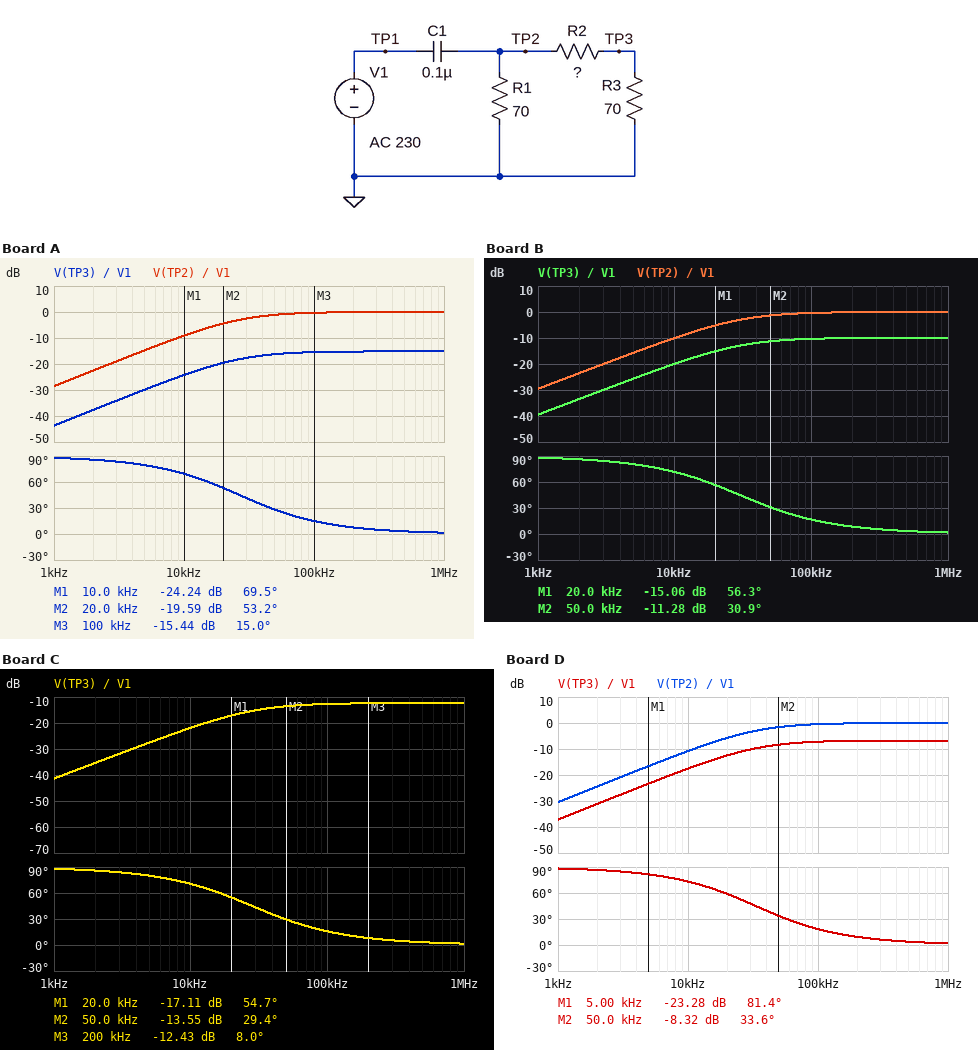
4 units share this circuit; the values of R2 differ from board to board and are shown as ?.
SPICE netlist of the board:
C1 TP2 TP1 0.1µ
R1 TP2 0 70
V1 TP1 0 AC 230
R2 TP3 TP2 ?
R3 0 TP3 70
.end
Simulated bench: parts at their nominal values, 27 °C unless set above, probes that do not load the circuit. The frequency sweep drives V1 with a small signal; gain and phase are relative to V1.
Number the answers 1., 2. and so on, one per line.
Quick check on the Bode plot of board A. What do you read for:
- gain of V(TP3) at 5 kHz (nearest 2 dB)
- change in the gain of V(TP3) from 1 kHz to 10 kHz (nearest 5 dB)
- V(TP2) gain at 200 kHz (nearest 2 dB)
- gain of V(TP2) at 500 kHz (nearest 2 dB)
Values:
1. -30 dB
2. 20 dB
3. 0 dB
4. 0 dB
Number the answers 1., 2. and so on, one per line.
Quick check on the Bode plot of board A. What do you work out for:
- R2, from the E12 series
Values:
1. 330 Ω
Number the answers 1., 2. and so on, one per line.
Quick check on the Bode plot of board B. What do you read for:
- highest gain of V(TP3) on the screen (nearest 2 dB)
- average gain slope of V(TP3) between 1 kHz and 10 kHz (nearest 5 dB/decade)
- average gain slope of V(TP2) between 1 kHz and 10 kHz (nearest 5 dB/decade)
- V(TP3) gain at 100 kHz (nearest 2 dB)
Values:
1. -10 dB
2. 20 dB/decade
3. 20 dB/decade
4. -10 dB
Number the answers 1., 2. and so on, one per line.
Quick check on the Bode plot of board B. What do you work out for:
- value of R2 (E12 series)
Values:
1. 150 Ω
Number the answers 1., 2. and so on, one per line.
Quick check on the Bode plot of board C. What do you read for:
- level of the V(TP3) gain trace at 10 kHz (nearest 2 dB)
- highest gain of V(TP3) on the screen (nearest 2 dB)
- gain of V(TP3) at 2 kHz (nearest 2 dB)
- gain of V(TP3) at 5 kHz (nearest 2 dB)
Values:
1. -22 dB
2. -12 dB
3. -36 dB
4. -28 dB
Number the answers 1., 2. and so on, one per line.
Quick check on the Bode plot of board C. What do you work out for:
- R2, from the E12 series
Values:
1. 220 Ω
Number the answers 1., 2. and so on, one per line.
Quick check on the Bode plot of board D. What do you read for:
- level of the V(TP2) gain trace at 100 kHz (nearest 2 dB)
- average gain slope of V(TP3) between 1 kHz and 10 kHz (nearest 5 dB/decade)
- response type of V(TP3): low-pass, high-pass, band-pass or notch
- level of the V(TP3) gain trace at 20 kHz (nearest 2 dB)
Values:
1. 0 dB
2. 20 dB/decade
3. high-pass
4. -12 dB
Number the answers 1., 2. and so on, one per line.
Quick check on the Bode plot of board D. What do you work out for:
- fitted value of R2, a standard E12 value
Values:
1. 82 Ω
